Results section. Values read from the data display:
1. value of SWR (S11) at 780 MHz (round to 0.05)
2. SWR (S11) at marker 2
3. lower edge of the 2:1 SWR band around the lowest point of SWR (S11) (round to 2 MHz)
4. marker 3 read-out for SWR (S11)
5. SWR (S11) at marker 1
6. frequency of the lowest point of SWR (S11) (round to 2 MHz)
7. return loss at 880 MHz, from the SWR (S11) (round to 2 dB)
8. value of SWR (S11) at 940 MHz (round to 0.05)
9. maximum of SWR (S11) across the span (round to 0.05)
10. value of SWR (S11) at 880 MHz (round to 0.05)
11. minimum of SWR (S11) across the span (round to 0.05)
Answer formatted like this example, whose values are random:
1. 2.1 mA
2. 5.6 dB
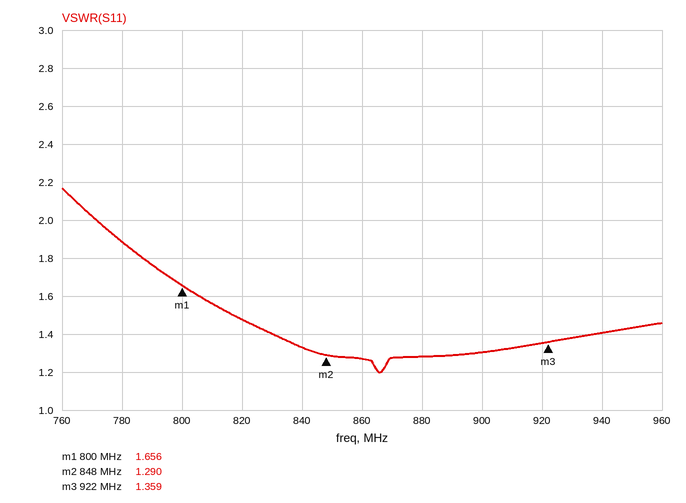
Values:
1. 1.90
2. 1.290
3. 772 MHz
4. 1.359
5. 1.656
6. 866 MHz
7. 18 dB
8. 1.40
9. 2.15
10. 1.30
11. 1.20
